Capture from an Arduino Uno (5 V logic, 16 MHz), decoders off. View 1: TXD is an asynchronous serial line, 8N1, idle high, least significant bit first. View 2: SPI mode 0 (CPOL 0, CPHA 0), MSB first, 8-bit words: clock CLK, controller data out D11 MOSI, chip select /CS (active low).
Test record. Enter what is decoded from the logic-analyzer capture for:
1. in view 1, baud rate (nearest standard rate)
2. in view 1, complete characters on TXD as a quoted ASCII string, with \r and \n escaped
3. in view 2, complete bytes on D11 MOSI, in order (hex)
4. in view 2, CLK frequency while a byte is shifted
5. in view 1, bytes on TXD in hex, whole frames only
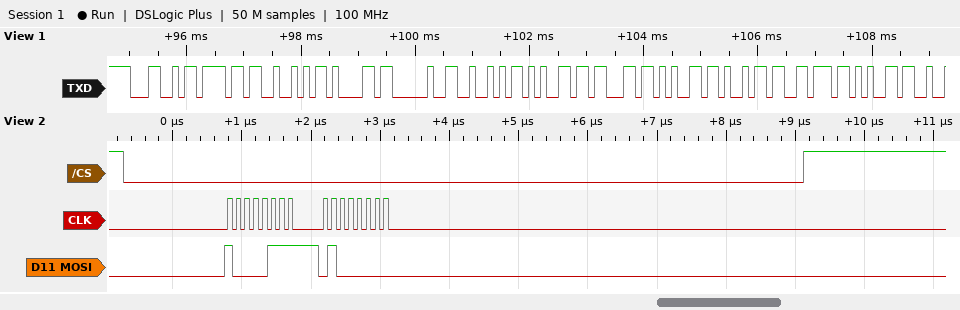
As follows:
9600 baud
"LoRa Receive"
87 40
8 MHz
0x4C 0x6F 0x52 0x61 0x20 0x52 0x65 0x63 0x65 0x69 0x76 0x65
